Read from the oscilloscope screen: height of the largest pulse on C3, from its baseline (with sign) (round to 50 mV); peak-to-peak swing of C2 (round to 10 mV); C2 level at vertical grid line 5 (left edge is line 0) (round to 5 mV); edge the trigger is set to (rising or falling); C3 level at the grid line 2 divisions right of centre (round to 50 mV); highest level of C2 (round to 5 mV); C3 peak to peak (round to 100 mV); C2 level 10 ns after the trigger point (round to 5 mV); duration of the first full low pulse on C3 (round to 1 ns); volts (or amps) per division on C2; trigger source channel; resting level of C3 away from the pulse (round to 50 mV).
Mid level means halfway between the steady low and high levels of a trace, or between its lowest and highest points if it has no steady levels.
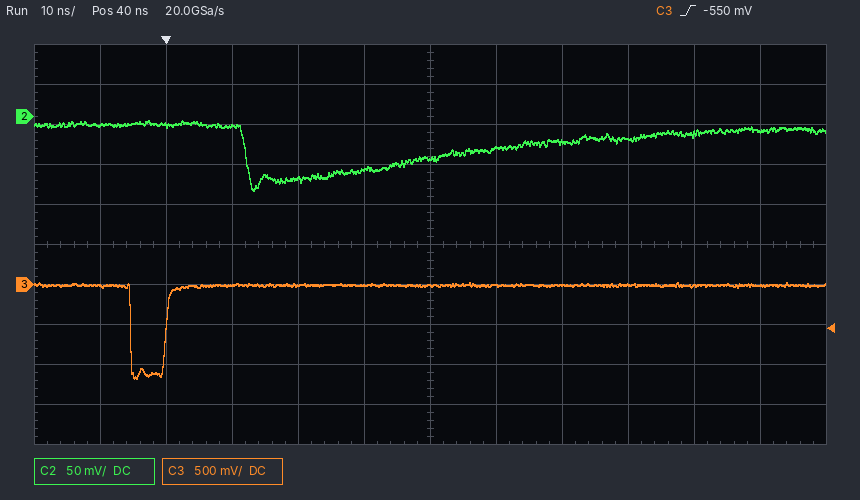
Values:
-1.15 V
90 mV
-65 mV
rising
0 mV
-5 mV
1.20 V
-10 mV
5 ns
50 mV
C3
0 mV
